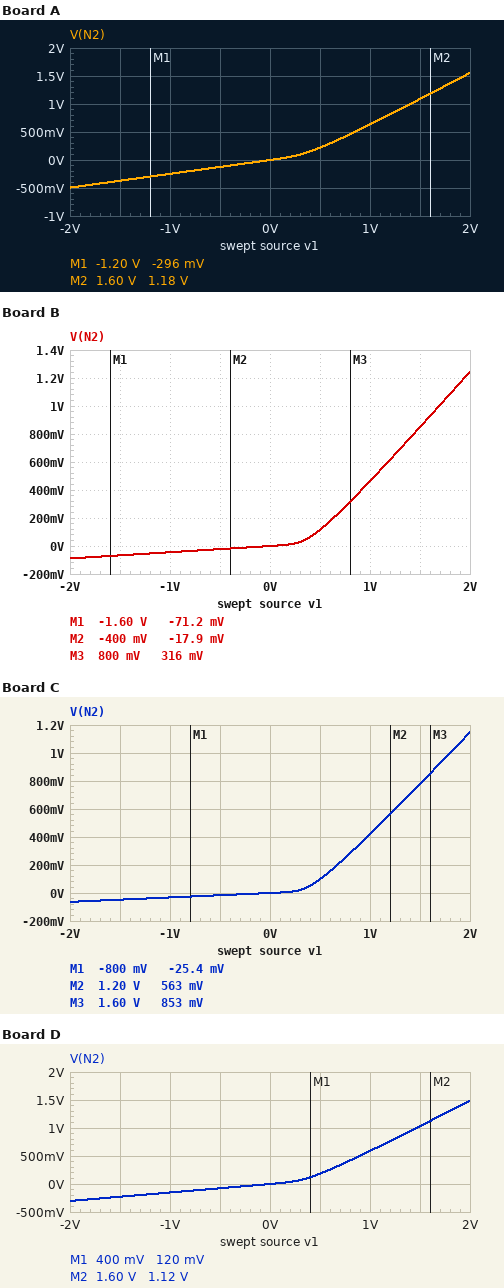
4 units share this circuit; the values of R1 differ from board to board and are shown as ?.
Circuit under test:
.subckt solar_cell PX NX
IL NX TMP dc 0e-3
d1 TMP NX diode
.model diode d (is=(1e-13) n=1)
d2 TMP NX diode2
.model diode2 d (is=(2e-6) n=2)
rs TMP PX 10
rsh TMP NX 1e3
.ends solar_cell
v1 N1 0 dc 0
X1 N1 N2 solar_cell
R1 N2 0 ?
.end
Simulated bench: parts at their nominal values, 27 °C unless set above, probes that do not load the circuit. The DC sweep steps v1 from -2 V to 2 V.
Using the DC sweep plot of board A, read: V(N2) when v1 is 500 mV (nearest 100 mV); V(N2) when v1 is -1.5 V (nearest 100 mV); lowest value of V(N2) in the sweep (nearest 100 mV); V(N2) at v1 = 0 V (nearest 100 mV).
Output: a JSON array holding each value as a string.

["200 mV", "-400 mV", "-500 mV", "0 V"]
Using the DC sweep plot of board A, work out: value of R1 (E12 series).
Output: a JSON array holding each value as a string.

["330 Ω"]
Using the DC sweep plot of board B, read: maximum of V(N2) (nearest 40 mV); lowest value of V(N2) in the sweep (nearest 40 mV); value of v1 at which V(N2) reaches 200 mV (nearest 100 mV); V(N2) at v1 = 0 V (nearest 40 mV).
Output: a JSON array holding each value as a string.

["1.24 V", "-80 mV", "600 mV", "0 V"]
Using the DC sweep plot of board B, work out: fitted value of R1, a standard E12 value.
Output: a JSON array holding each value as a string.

["47 Ω"]
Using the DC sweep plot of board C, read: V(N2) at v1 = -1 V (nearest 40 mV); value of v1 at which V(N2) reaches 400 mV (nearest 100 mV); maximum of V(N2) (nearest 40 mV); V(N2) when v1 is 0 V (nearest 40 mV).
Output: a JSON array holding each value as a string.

["-40 mV", "1.0 V", "1.16 V", "0 V"]
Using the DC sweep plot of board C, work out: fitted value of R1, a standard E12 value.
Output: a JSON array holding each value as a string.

["33 Ω"]
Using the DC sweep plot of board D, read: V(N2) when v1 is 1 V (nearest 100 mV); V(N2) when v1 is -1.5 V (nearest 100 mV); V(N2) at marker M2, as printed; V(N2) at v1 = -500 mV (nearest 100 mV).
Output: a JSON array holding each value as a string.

["600 mV", "-200 mV", "1.12 V", "-100 mV"]
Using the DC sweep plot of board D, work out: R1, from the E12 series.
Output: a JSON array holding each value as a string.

["180 Ω"]
